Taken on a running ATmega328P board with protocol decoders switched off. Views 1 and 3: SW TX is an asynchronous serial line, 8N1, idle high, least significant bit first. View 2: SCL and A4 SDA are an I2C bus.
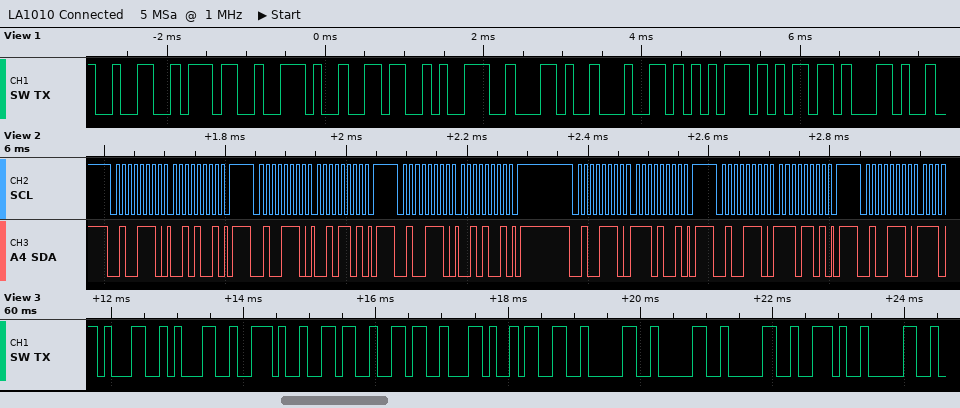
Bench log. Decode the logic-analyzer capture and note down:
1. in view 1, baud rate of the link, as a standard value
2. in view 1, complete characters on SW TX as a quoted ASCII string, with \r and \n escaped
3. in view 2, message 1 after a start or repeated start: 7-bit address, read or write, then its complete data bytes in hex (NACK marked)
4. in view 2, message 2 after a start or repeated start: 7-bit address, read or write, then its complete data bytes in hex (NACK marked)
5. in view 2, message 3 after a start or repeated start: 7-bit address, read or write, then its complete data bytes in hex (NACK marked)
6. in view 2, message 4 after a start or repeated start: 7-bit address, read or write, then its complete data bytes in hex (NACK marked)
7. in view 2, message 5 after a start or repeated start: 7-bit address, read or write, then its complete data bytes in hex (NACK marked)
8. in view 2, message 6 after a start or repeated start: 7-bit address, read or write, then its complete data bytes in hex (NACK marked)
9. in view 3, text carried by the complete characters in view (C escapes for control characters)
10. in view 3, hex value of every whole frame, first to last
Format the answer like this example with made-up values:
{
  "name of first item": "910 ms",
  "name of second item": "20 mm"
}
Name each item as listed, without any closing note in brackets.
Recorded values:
{
  "in view 1, baud rate of the link, as a standard value": "9600 baud",
  "in view 1, complete characters on SW TX as a quoted ASCII string, with \\r and \\n escaped": "\"27.69,dum,\"",
  "in view 2, message 1 after a start or repeated start: 7-bit address, read or write, then its complete data bytes in hex": "0x27 write: 29",
  "in view 2, message 2 after a start or repeated start: 7-bit address, read or write, then its complete data bytes in hex": "0x27 write: 2D",
  "in view 2, message 3 after a start or repeated start: 7-bit address, read or write, then its complete data bytes in hex": "0x27 write: 29",
  "in view 2, message 4 after a start or repeated start: 7-bit address, read or write, then its complete data bytes in hex": "0x27 write: E9",
  "in view 2, message 5 after a start or repeated start: 7-bit address, read or write, then its complete data bytes in hex": "0x27 write: ED",
  "in view 2, message 6 after a start or repeated start: 7-bit address, read or write, then its complete data bytes in hex": "0x27 write",
  "in view 3, text carried by the complete characters in view": "\"11.66,3000.0\"",
  "in view 3, hex value of every whole frame, first to last": "0x31 0x31 0x2E 0x36 0x36 0x2C 0x33 0x30 0x30 0x30 0x2E 0x30"
}
